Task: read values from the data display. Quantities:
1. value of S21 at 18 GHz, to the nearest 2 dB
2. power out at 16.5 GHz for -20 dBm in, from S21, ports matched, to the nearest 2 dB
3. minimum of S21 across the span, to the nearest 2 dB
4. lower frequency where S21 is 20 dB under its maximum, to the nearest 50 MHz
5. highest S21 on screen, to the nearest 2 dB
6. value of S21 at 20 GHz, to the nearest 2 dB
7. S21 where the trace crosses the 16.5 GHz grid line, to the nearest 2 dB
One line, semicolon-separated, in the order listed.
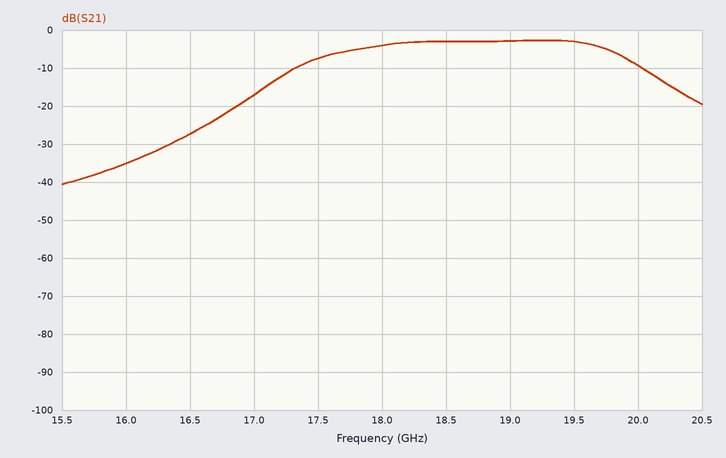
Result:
-4 dB; -48 dBm; -40 dB; 16.75 GHz; -2 dB; -10 dB; -28 dB
